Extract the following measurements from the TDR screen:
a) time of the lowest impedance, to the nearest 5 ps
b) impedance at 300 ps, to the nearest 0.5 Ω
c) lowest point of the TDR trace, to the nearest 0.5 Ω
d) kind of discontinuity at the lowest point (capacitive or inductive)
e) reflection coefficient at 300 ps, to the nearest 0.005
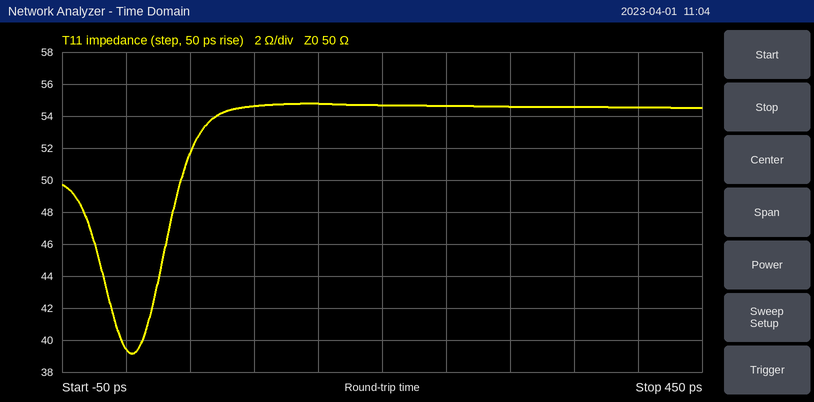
5 ps
54.5 Ω
39.0 Ω
capacitive
+0.045
